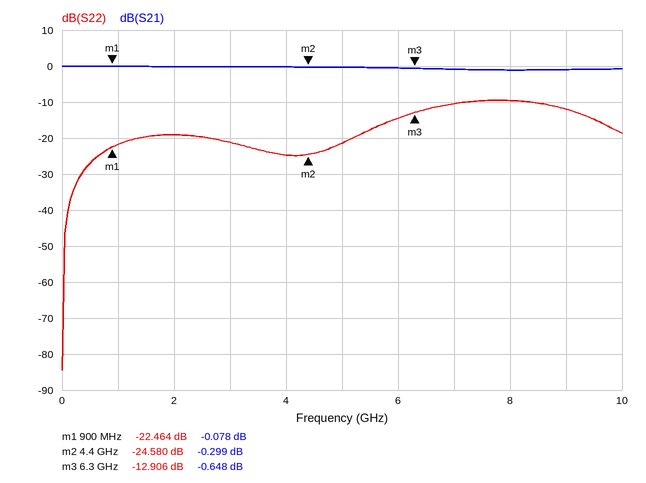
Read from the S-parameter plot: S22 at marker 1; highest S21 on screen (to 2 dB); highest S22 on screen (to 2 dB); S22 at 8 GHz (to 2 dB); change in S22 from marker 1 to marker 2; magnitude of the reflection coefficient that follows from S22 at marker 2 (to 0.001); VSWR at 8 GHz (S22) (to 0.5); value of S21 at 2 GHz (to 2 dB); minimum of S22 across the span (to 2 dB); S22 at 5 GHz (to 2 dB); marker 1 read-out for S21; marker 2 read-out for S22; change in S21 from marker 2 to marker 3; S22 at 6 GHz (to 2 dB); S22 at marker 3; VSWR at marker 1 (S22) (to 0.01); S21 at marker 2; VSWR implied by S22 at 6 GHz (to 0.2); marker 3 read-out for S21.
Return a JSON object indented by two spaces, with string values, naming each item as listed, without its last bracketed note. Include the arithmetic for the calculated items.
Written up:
{
  "S22 at marker 1": "-22.464 dB",
  "highest S21 on screen": "0 dB",
  "highest S22 on screen": "-10 dB",
  "S22 at 8 GHz": "-10 dB",
  "change in S22 from marker 1 to marker 2": "-24.58 − (-22.464) = -2.116 dB",
  "magnitude of the reflection coefficient that follows from S22 at marker 2": "10^(-24.58/20) ≈ 0.059",
  "VSWR at 8 GHz (S22)": "|Γ| = 10^(-10/20) = 0.3162; VSWR = (1 + 0.3162)/(1 − 0.3162) ≈ 1.92, so 2.0 to the nearest 0.5",
  "value of S21 at 2 GHz": "0 dB",
  "minimum of S22 across the span": "-84 dB",
  "S22 at 5 GHz": "-22 dB",
  "marker 1 read-out for S21": "-0.078 dB",
  "marker 2 read-out for S22": "-24.580 dB",
  "change in S21 from marker 2 to marker 3": "-0.648 − (-0.299) = -0.349 dB",
  "S22 at 6 GHz": "-14 dB",
  "S22 at marker 3": "-12.906 dB",
  "VSWR at marker 1 (S22)": "(1 + 0.0753)/(1 − 0.0753) ≈ 1.16",
  "S21 at marker 2": "-0.299 dB",
  "VSWR implied by S22 at 6 GHz": "|Γ| = 10^(-14/20) = 0.1995; VSWR = (1 + 0.1995)/(1 − 0.1995) ≈ 1.50, so 1.4 to the nearest 0.2",
  "marker 3 read-out for S21": "-0.648 dB"
}
